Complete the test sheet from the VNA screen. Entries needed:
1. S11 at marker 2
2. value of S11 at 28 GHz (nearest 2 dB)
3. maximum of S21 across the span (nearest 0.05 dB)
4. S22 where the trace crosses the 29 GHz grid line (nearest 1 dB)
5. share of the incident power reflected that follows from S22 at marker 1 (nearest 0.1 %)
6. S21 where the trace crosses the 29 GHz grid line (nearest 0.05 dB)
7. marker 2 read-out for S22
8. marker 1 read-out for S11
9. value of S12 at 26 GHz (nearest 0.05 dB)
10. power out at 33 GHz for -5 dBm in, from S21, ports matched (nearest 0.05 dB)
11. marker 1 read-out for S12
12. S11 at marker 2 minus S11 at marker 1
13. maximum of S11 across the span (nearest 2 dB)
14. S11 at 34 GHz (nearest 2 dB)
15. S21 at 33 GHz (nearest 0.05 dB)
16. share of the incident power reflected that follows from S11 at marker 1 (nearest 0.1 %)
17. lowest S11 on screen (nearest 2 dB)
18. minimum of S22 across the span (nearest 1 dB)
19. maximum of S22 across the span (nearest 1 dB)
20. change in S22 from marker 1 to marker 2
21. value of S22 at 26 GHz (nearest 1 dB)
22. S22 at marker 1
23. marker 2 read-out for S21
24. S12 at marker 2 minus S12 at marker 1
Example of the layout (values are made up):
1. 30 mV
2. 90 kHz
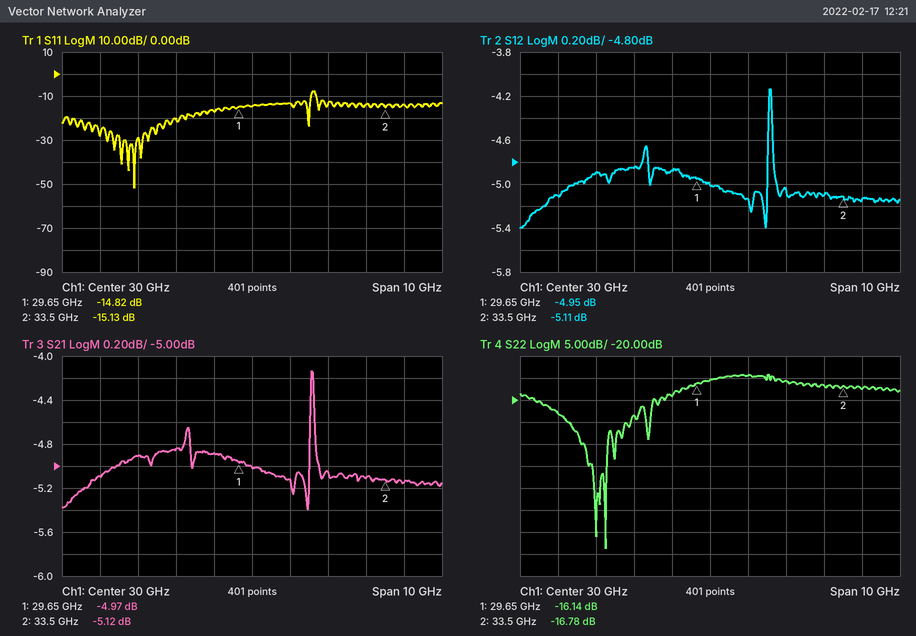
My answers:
1. -15.13 dB
2. -20 dB
3. -4.15 dB
4. -19 dB
5. 2.4 %
6. -4.90 dB
7. -16.78 dB
8. -14.82 dB
9. -5.10 dB
10. -10.10 dBm
11. -4.95 dB
12. -0.31 dB
13. -8 dB
14. -14 dB
15. -5.10 dB
16. 3.3 %
17. -52 dB
18. -54 dB
19. -14 dB
20. -0.64 dB
21. -23 dB
22. -16.14 dB
23. -5.12 dB
24. -0.16 dB
